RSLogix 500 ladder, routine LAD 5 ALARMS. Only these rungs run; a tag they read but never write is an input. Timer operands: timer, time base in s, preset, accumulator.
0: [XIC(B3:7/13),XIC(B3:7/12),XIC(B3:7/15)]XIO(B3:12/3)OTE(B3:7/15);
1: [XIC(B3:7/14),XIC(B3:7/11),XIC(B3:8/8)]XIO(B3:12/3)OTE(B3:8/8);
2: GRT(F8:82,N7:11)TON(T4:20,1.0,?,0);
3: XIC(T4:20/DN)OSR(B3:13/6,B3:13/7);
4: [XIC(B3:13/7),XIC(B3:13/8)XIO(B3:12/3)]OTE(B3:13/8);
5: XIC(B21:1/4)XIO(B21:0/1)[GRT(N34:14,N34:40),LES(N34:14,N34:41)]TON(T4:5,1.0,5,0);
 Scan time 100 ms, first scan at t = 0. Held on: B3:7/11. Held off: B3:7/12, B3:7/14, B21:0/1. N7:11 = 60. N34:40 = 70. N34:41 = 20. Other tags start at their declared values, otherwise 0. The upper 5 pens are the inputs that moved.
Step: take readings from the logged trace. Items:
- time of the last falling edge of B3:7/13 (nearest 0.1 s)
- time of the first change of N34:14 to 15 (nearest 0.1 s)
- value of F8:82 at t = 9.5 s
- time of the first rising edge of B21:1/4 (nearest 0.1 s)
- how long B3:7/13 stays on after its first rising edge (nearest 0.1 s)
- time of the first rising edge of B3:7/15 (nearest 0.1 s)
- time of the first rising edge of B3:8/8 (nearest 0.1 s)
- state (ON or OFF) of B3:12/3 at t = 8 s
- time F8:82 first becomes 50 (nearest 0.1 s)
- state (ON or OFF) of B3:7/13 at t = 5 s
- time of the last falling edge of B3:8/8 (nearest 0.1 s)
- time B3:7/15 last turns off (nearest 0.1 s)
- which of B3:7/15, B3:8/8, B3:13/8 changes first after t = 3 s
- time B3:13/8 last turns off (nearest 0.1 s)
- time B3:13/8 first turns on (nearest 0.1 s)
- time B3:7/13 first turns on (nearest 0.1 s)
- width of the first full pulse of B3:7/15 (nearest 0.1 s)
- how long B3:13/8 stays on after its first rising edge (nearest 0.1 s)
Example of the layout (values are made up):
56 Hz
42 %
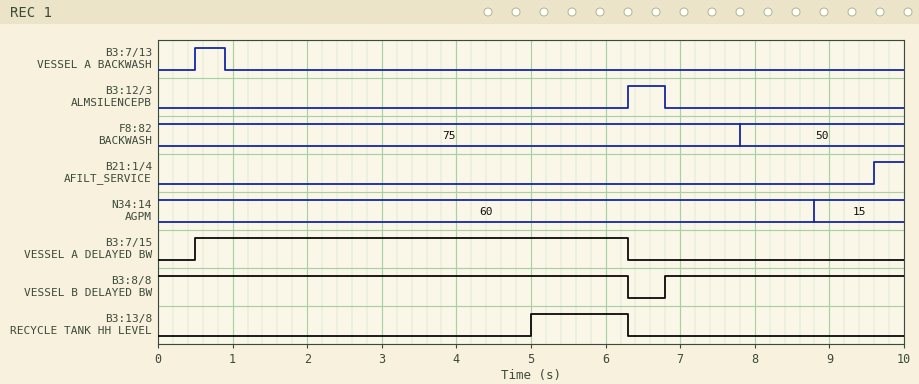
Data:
0.9 s
8.8 s
50
9.6 s
0.4 s
0.5 s
6.8 s
OFF
7.8 s
OFF
6.3 s
6.3 s
B3:13/8
6.3 s
5.0 s
0.5 s
5.8 s
1.3 s
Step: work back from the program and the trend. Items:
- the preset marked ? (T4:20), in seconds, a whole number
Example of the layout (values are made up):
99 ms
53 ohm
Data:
5 s
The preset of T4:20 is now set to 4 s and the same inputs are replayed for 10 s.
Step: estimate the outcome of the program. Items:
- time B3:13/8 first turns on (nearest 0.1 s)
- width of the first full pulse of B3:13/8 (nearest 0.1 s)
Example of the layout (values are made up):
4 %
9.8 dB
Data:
4.0 s
2.3 s
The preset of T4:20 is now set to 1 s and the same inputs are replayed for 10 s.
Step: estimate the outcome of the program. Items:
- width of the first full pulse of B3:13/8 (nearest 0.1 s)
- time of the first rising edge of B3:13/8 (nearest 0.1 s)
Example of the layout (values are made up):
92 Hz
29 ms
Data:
5.3 s
1.0 s
